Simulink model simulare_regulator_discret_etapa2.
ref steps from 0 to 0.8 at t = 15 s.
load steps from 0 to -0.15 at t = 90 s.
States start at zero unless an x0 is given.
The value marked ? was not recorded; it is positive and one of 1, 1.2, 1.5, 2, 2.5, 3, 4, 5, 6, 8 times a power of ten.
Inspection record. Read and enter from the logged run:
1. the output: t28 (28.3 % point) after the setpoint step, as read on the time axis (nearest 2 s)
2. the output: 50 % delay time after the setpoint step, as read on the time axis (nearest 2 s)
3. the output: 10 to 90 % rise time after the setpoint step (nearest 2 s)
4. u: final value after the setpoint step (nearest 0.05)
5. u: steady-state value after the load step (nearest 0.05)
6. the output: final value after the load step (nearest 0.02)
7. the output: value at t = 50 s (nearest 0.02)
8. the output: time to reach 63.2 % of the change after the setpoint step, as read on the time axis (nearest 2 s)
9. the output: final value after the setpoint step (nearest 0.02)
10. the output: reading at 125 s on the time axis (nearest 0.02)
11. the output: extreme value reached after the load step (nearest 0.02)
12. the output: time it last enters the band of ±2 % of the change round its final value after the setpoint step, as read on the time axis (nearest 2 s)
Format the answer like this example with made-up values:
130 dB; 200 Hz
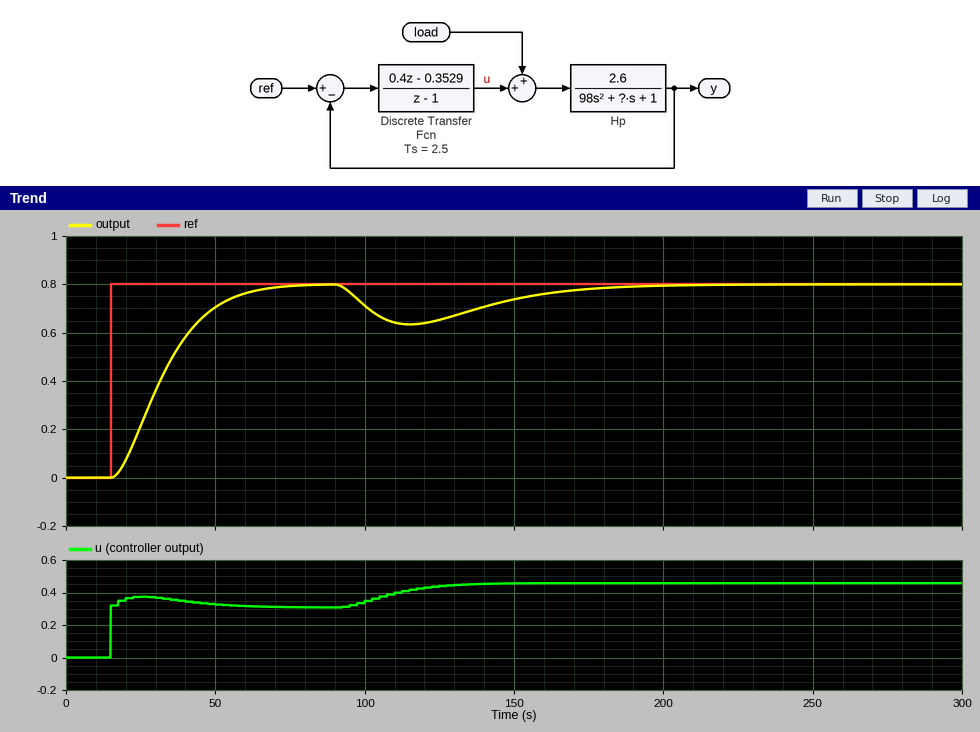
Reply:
26 s; 32 s; 32 s; 0.30; 0.45; 0.80; 0.70; 36 s; 0.80; 0.66; 0.64; 68 s
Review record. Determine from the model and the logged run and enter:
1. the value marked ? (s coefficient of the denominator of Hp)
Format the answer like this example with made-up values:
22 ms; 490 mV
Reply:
25
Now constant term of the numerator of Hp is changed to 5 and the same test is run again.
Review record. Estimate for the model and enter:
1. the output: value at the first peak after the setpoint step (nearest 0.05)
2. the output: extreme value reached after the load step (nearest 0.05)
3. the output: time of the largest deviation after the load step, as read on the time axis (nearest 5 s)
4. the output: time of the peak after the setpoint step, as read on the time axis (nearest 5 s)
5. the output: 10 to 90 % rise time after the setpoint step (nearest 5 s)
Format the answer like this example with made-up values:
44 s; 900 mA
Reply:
0.85; 0.55; 110 s; 45 s; 15 s
